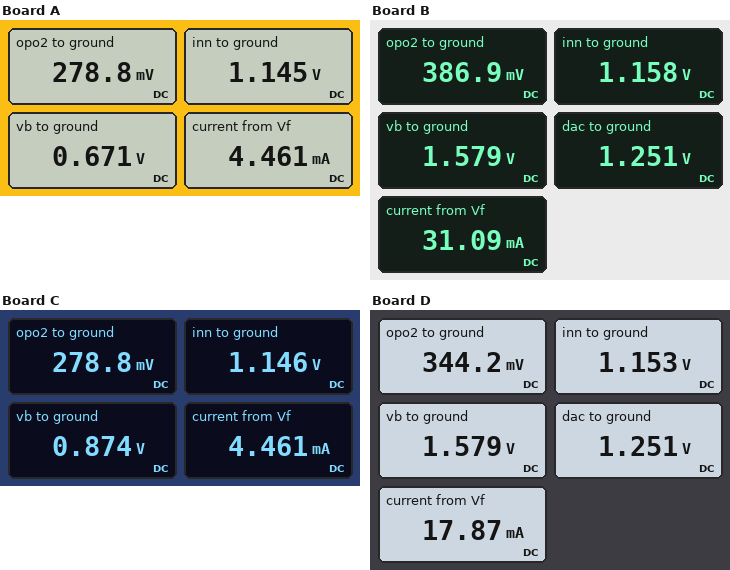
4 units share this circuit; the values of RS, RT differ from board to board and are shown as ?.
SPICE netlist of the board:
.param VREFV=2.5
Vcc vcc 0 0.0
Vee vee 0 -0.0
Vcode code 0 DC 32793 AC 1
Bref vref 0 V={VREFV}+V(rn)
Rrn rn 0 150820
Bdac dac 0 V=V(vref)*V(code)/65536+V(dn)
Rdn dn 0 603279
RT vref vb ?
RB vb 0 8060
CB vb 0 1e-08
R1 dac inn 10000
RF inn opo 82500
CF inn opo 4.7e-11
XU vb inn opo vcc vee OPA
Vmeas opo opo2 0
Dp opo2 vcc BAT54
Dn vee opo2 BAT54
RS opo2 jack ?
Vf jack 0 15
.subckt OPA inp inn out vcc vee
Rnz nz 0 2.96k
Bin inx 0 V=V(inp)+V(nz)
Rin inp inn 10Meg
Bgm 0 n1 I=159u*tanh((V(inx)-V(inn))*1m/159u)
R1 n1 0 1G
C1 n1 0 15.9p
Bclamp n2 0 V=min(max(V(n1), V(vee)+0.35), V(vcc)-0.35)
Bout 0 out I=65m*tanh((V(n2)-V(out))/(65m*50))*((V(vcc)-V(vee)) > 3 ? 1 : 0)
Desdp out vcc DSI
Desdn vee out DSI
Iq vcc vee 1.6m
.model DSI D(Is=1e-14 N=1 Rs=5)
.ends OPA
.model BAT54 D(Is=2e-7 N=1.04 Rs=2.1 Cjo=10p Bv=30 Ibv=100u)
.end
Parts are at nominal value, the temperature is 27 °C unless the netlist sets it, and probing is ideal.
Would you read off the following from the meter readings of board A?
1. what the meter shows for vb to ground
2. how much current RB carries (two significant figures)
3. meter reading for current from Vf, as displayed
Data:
0.671 V
83 µA
4.461 mA
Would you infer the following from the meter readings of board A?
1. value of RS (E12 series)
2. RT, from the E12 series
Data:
3.3 kΩ
22 kΩ
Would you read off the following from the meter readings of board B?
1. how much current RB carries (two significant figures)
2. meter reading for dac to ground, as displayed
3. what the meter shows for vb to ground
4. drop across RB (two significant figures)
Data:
200 µA
1.251 V
1.579 V
1.6 V
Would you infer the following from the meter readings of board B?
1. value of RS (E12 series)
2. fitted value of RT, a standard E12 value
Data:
470 Ω
4.7 kΩ
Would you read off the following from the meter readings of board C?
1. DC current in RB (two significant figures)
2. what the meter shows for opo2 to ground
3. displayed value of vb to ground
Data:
110 µA
278.8 mV
0.874 V
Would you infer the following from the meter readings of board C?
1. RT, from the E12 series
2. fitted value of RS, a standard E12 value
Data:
15 kΩ
3.3 kΩ
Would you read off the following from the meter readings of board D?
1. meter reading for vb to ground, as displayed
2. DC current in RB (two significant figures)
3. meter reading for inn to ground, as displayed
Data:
1.579 V
200 µA
1.153 V
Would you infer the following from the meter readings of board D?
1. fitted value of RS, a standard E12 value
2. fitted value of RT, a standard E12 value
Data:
820 Ω
4.7 kΩ
